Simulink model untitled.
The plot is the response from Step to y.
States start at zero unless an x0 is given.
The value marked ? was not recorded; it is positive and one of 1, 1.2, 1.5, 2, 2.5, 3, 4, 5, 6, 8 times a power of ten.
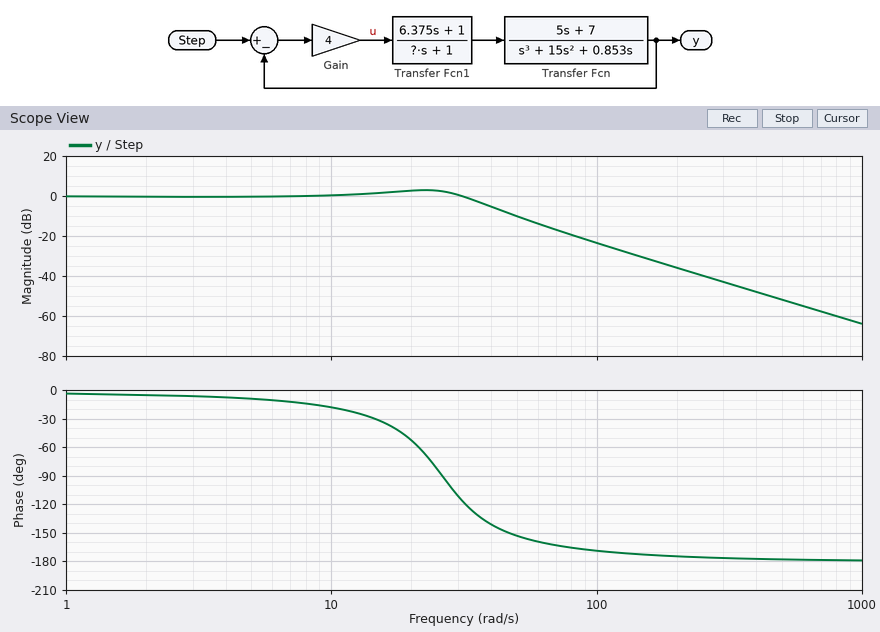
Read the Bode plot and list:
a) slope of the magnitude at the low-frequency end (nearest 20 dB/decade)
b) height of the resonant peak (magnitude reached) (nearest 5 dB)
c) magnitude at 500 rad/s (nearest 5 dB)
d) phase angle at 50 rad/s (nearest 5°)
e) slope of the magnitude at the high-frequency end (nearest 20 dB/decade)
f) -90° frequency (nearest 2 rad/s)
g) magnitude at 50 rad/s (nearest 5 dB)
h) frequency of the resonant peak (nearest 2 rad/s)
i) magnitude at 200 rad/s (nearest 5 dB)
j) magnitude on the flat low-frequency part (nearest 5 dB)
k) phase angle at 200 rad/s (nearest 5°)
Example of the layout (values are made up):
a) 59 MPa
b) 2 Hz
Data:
a) 0 dB/decade
b) 5 dB
c) -50 dB
d) -155°
e) -40 dB/decade
f) 26 rad/s
g) -10 dB
h) 22 rad/s
i) -35 dB
j) 0 dB
k) -175°
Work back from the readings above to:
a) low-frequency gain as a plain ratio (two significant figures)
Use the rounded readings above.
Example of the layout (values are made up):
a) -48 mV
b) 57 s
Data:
a) 1.0
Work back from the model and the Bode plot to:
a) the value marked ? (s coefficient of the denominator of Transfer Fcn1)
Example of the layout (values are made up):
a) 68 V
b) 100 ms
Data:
a) 0.2
